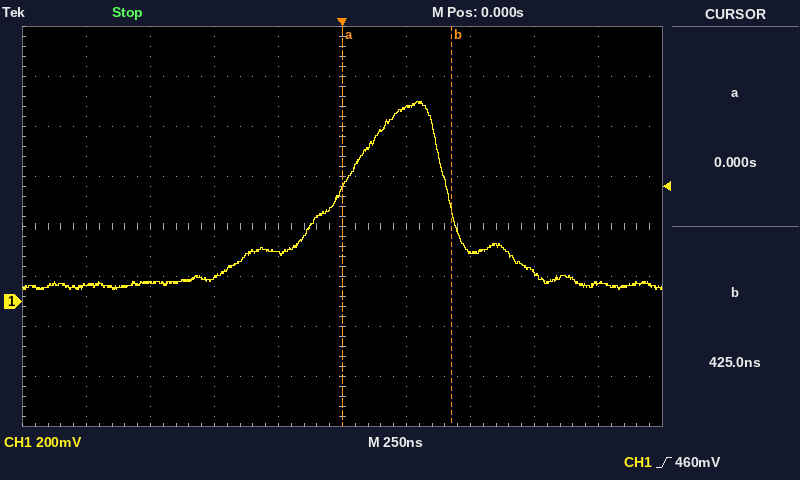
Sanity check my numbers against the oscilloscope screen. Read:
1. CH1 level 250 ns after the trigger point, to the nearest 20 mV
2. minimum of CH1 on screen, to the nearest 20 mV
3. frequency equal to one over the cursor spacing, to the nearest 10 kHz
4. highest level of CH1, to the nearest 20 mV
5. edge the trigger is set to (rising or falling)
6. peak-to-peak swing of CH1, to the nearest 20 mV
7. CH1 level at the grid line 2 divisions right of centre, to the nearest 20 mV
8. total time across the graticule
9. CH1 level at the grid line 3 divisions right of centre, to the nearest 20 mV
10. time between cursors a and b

780 mV
40 mV
2.35 MHz
800 mV
rising
760 mV
200 mV
2.5 µs
120 mV
425 ns
